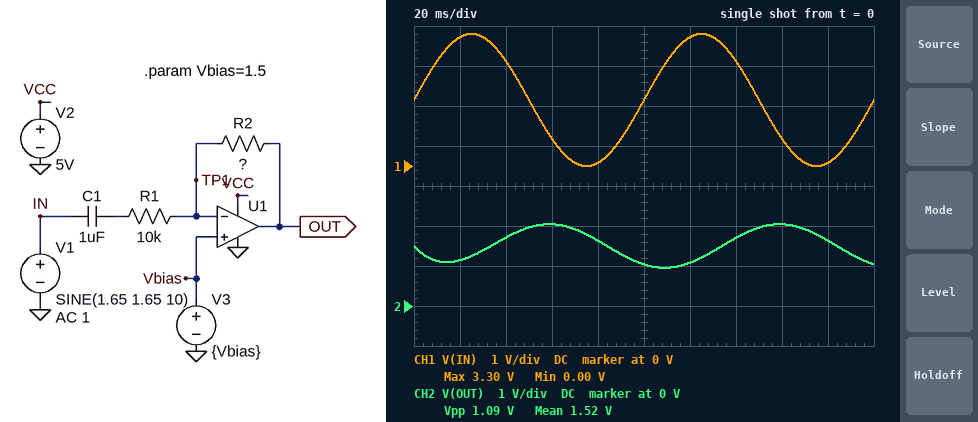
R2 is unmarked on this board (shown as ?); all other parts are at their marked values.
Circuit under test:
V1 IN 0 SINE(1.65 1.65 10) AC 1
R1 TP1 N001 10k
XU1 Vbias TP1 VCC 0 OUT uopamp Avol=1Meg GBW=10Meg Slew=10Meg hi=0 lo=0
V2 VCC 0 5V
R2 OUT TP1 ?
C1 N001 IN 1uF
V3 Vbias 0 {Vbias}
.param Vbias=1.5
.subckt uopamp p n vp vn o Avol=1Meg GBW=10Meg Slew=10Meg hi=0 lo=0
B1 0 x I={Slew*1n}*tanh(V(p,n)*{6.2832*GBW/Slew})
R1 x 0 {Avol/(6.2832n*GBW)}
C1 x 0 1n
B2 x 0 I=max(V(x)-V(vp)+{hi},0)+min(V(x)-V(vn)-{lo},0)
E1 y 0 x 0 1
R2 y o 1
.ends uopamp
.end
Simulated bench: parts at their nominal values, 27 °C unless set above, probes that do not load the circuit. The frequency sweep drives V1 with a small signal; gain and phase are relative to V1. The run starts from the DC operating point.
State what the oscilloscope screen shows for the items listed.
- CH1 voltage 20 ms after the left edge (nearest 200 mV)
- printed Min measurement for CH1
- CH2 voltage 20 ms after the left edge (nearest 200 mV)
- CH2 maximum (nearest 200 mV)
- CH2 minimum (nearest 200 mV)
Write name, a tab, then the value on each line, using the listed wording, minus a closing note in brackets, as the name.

CH1 voltage 20 ms after the left edge	3.2 V
printed Min measurement for CH1	0.00 V
CH2 voltage 20 ms after the left edge	1.2 V
CH2 maximum	2.0 V
CH2 minimum	1.0 V
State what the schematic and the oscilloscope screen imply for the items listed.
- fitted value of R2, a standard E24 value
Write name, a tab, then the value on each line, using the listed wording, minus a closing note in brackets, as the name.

fitted value of R2, a standard E24 value	6.2 kΩ
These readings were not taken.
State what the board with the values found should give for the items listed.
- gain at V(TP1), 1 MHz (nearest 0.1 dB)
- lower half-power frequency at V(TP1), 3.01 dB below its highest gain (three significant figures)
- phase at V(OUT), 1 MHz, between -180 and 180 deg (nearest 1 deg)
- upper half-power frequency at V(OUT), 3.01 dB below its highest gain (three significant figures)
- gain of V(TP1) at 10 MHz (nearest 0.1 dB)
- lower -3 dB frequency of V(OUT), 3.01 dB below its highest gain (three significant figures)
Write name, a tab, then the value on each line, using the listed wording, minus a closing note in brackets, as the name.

gain at V(TP1), 1 MHz	-24.3 dB
lower half-power frequency at V(TP1), 3.01 dB below its highest gain	6.17 MHz
phase at V(OUT), 1 MHz, between -180 and 180 deg	171 deg
upper half-power frequency at V(OUT), 3.01 dB below its highest gain	6.17 MHz
gain of V(TP1) at 10 MHz	-9.7 dB
lower -3 dB frequency of V(OUT), 3.01 dB below its highest gain	15.9 Hz
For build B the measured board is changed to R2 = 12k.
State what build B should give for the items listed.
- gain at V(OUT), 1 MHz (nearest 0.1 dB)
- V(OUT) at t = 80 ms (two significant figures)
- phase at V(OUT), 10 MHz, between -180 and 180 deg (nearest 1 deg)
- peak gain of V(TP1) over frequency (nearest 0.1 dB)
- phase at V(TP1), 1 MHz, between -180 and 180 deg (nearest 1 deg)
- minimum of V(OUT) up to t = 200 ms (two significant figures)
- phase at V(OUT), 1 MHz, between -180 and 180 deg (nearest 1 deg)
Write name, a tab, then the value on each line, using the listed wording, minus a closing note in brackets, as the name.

gain at V(OUT), 1 MHz	1.4 dB
V(OUT) at t = 80 ms	1.8 V
phase at V(OUT), 10 MHz, between -180 and 180 deg	114 deg
peak gain of V(TP1) over frequency	-5.3 dB
phase at V(TP1), 1 MHz, between -180 and 180 deg	78 deg
minimum of V(OUT) up to t = 200 ms	450 mV
phase at V(OUT), 1 MHz, between -180 and 180 deg	168 deg
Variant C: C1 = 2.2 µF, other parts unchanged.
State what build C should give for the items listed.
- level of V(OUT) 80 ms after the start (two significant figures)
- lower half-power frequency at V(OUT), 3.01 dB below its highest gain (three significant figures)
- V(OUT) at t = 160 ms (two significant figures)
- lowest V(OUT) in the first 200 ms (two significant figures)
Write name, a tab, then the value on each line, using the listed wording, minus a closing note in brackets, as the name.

level of V(OUT) 80 ms after the start	2.0 V
lower half-power frequency at V(OUT), 3.01 dB below its highest gain	7.23 Hz
V(OUT) at t = 160 ms	2.3 V
lowest V(OUT) in the first 200 ms	670 mV
